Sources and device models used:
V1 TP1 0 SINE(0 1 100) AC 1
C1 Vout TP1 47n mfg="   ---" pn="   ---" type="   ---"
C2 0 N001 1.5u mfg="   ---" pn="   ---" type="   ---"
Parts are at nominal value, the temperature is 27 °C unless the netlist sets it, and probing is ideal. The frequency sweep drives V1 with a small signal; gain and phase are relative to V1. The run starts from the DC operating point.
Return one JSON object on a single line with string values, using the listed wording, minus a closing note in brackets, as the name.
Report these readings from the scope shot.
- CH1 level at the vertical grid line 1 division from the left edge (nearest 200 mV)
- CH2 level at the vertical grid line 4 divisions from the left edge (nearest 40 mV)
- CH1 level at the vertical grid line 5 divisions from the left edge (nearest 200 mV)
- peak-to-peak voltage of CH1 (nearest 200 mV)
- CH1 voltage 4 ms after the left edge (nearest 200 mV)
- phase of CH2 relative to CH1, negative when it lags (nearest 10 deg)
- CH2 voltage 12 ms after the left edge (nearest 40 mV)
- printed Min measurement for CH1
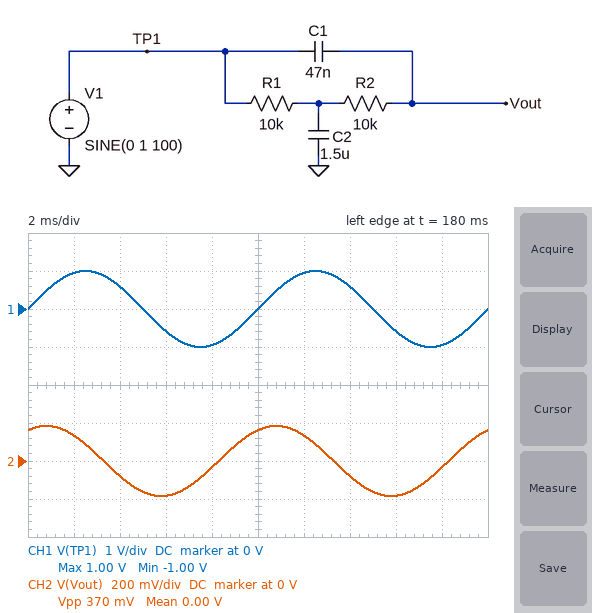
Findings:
{"CH1 level at the vertical grid line 1 division from the left edge": "1.0 V", "CH2 level at the vertical grid line 4 divisions from the left edge": "-40 mV", "CH1 level at the vertical grid line 5 divisions from the left edge": "0 V", "peak-to-peak voltage of CH1": "2.0 V", "CH1 voltage 4 ms after the left edge": "600 mV", "phase of CH2 relative to CH1, negative when it lags": "60 deg", "CH2 voltage 12 ms after the left edge": "120 mV", "printed Min measurement for CH1": "-1.00 V"}
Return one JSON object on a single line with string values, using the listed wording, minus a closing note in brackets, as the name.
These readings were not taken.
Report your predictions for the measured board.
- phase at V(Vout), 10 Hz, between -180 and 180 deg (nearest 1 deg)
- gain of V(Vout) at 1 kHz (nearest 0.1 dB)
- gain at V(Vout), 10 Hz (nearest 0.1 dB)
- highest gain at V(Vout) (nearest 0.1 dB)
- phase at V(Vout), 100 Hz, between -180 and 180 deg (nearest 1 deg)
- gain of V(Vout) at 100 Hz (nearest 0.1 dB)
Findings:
{"phase at V(Vout), 10 Hz, between -180 and 180 deg": "-42 deg", "gain of V(Vout) at 1 kHz": "-0.5 dB", "gain at V(Vout), 10 Hz": "-3.1 dB", "highest gain at V(Vout)": "0 dB", "phase at V(Vout), 100 Hz, between -180 and 180 deg": "62 deg", "gain of V(Vout) at 100 Hz": "-14.7 dB"}
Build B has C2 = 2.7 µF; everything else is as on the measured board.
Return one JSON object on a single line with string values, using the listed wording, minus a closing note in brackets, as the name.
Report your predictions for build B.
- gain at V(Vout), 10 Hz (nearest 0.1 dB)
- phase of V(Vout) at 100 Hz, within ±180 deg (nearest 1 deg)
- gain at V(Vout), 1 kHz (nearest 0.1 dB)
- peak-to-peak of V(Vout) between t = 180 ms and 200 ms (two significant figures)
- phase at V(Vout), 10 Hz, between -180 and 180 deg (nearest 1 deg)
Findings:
{"gain at V(Vout), 10 Hz": "-6.4 dB", "phase of V(Vout) at 100 Hz, within ±180 deg": "69 deg", "gain at V(Vout), 1 kHz": "-0.5 dB", "peak-to-peak of V(Vout) between t = 180 ms and 200 ms": "450 mV", "phase at V(Vout), 10 Hz, between -180 and 180 deg": "-58 deg"}
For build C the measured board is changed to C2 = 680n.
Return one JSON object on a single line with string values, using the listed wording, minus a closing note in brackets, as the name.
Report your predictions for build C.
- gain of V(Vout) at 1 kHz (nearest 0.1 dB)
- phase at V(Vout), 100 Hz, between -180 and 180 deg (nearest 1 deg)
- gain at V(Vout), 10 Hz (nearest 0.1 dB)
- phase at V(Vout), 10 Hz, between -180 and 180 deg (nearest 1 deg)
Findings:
{"gain of V(Vout) at 1 kHz": "-0.6 dB", "phase at V(Vout), 100 Hz, between -180 and 180 deg": "21 deg", "gain at V(Vout), 10 Hz": "-0.9 dB", "phase at V(Vout), 10 Hz, between -180 and 180 deg": "-23 deg"}
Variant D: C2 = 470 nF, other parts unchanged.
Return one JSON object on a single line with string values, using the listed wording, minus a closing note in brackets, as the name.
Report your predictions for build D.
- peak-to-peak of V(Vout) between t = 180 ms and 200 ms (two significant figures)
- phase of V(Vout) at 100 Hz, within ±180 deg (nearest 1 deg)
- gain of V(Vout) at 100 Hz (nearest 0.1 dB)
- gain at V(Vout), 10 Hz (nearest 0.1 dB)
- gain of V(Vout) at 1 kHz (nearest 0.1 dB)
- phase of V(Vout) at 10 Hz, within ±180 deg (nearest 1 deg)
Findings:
{"peak-to-peak of V(Vout) between t = 180 ms and 200 ms": "340 mV", "phase of V(Vout) at 100 Hz, within ±180 deg": "-10 deg", "gain of V(Vout) at 100 Hz": "-15.4 dB", "gain at V(Vout), 10 Hz": "-0.5 dB", "gain of V(Vout) at 1 kHz": "-0.7 dB", "phase of V(Vout) at 10 Hz, within ±180 deg": "-16 deg"}
